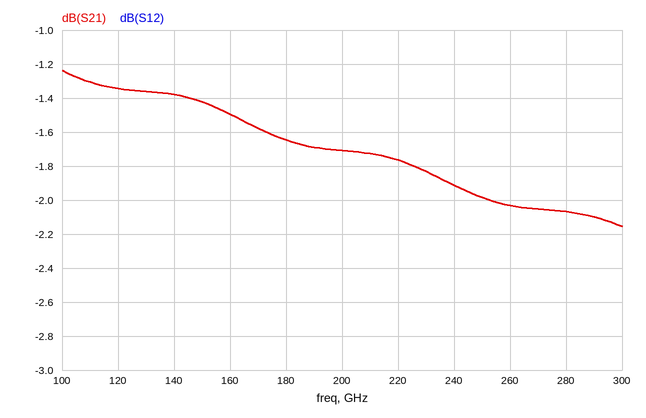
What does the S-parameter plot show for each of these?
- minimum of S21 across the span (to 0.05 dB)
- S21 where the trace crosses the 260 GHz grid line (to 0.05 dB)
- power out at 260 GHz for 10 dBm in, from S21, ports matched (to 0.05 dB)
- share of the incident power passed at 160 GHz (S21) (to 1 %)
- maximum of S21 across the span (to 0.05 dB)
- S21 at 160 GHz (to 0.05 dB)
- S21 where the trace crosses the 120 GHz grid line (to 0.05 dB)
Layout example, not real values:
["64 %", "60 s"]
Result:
["-2.15 dB", "-2.05 dB", "7.95 dBm", "71 %", "-1.25 dB", "-1.50 dB", "-1.35 dB"]
